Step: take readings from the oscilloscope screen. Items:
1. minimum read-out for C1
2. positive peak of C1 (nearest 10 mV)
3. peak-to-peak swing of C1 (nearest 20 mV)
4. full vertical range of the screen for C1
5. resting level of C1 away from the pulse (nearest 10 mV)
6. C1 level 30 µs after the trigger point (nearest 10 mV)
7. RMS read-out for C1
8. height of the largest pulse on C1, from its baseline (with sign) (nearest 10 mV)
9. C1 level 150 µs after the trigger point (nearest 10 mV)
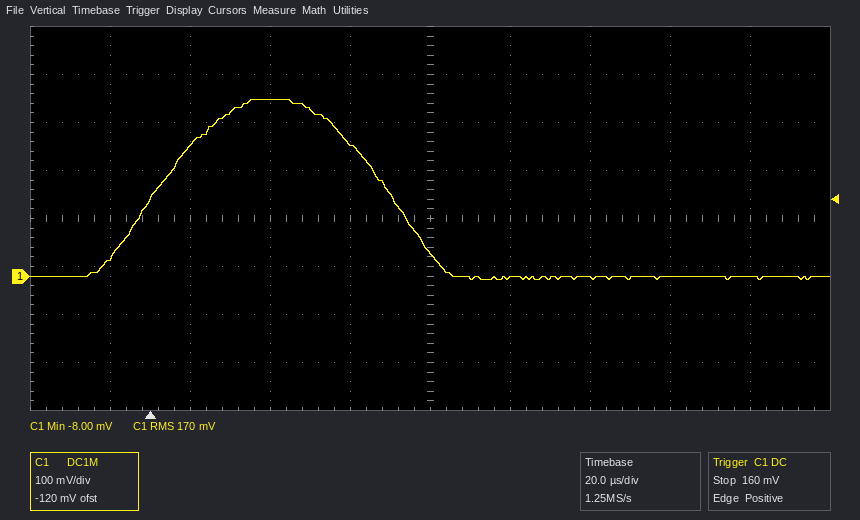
-8.00 mV
370 mV
380 mV
800 mV
0 mV
370 mV
170 mV
+370 mV
0 mV
